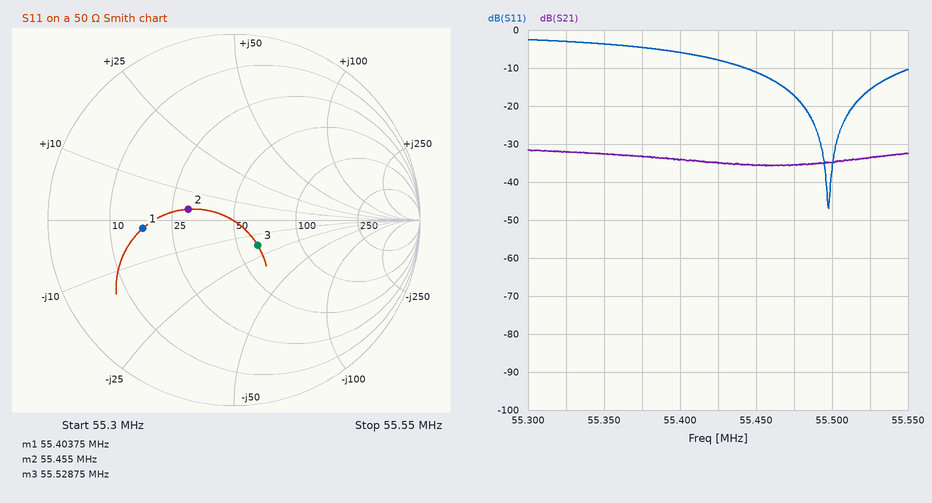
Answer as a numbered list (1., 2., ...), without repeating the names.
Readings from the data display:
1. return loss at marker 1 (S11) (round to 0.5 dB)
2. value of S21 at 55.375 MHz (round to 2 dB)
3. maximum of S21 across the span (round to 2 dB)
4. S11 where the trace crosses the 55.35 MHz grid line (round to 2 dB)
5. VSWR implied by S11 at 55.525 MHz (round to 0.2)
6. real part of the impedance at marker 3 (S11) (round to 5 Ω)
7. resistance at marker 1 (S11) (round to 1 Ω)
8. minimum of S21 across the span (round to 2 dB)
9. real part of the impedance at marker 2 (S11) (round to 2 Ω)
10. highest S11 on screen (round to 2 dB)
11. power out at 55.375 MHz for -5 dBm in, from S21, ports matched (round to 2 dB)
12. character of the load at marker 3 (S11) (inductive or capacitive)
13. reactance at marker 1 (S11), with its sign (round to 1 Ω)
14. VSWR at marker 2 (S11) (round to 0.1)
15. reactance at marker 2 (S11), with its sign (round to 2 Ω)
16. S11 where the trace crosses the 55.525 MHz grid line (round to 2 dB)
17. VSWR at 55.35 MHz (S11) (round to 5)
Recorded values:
1. 6.0 dB
2. -34 dB
3. -32 dB
4. -4 dB
5. 1.4
6. 60 Ω
7. 17 Ω
8. -36 dB
9. 30 Ω
10. -2 dB
11. -38 dBm
12. capacitive
13. -2 Ω
14. 1.7
15. +4 Ω
16. -16 dB
17. 5
